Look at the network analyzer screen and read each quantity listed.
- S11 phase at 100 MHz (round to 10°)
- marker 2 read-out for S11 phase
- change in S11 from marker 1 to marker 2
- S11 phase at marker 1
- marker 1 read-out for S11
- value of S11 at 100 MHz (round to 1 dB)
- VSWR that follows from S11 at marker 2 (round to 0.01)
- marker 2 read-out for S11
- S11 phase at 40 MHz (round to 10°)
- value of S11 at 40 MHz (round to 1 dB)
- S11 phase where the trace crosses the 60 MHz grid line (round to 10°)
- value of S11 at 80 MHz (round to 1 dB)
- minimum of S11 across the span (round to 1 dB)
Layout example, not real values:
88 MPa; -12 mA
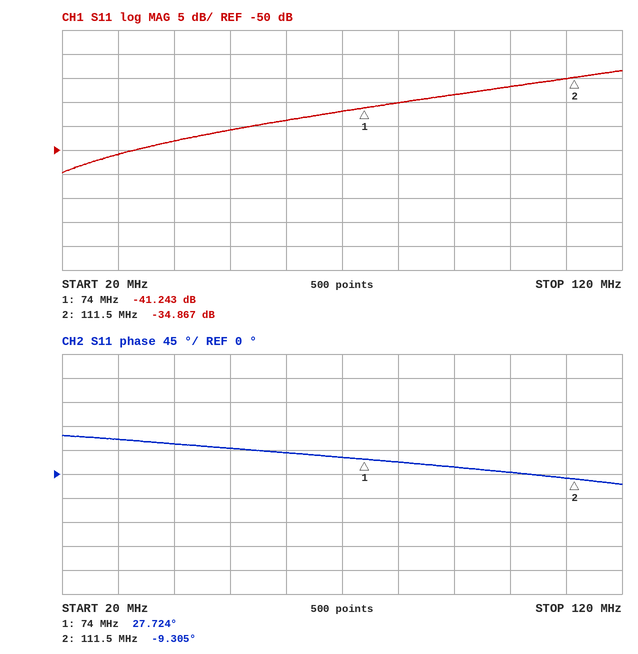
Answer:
0°; -9.305°; 6.376 dB; 27.724°; -41.243 dB; -37 dB; 1.04; -34.867 dB; 60°; -48 dB; 40°; -40 dB; -55 dB
